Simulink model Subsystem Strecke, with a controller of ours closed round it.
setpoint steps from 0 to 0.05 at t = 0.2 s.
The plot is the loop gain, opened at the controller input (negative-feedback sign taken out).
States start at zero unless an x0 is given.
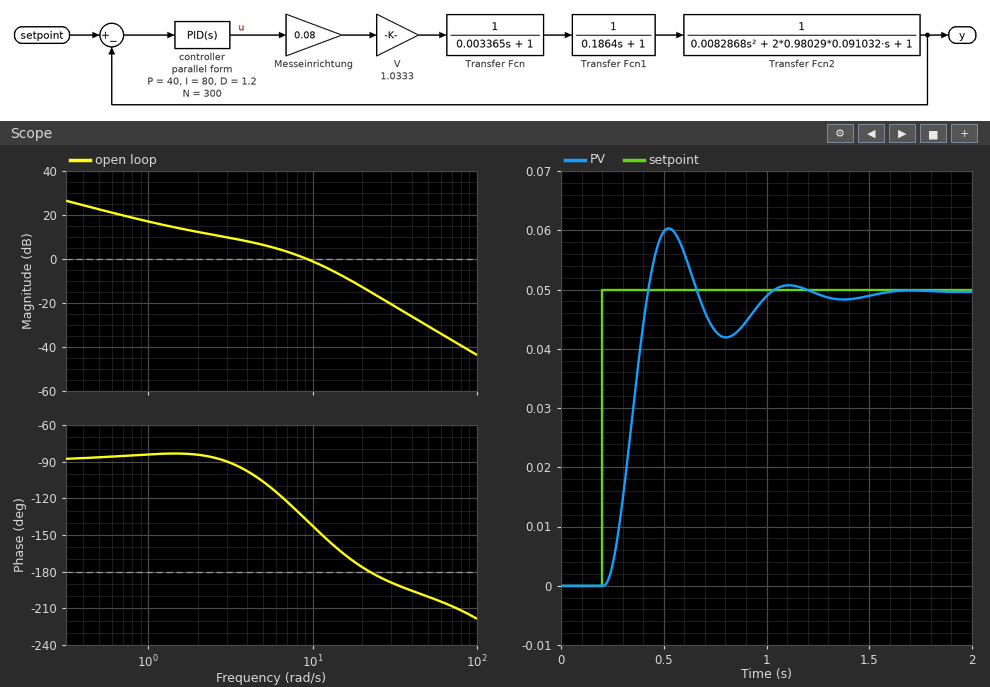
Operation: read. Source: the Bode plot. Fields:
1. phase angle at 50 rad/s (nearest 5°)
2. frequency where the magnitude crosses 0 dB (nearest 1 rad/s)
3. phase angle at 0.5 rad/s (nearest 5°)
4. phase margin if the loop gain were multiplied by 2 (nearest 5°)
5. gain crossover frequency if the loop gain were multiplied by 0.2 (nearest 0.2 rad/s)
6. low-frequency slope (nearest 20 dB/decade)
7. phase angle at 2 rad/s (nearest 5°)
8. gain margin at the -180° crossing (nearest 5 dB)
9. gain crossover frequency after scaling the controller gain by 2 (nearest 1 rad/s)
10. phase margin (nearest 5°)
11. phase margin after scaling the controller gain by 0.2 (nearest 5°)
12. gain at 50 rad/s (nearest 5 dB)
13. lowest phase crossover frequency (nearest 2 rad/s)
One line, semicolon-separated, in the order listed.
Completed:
-200°; 9 rad/s; -85°; 20°; 1.6 rad/s; -20 dB/decade; -85°; 15 dB; 14 rad/s; 40°; 95°; -30 dB; 22 rad/s
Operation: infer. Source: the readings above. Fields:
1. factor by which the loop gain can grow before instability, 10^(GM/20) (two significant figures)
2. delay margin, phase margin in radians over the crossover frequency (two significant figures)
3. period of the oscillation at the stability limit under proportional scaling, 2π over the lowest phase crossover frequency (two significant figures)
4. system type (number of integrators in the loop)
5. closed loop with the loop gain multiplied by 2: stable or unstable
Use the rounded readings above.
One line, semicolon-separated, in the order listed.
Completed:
5.6; 0.078 s; 0.29 s; 1; stable
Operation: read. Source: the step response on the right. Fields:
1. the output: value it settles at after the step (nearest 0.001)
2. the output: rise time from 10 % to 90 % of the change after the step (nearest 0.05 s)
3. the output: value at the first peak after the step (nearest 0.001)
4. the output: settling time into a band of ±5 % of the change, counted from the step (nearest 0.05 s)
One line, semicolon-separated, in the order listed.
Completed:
0.050; 0.15 s; 0.060; 0.75 s
